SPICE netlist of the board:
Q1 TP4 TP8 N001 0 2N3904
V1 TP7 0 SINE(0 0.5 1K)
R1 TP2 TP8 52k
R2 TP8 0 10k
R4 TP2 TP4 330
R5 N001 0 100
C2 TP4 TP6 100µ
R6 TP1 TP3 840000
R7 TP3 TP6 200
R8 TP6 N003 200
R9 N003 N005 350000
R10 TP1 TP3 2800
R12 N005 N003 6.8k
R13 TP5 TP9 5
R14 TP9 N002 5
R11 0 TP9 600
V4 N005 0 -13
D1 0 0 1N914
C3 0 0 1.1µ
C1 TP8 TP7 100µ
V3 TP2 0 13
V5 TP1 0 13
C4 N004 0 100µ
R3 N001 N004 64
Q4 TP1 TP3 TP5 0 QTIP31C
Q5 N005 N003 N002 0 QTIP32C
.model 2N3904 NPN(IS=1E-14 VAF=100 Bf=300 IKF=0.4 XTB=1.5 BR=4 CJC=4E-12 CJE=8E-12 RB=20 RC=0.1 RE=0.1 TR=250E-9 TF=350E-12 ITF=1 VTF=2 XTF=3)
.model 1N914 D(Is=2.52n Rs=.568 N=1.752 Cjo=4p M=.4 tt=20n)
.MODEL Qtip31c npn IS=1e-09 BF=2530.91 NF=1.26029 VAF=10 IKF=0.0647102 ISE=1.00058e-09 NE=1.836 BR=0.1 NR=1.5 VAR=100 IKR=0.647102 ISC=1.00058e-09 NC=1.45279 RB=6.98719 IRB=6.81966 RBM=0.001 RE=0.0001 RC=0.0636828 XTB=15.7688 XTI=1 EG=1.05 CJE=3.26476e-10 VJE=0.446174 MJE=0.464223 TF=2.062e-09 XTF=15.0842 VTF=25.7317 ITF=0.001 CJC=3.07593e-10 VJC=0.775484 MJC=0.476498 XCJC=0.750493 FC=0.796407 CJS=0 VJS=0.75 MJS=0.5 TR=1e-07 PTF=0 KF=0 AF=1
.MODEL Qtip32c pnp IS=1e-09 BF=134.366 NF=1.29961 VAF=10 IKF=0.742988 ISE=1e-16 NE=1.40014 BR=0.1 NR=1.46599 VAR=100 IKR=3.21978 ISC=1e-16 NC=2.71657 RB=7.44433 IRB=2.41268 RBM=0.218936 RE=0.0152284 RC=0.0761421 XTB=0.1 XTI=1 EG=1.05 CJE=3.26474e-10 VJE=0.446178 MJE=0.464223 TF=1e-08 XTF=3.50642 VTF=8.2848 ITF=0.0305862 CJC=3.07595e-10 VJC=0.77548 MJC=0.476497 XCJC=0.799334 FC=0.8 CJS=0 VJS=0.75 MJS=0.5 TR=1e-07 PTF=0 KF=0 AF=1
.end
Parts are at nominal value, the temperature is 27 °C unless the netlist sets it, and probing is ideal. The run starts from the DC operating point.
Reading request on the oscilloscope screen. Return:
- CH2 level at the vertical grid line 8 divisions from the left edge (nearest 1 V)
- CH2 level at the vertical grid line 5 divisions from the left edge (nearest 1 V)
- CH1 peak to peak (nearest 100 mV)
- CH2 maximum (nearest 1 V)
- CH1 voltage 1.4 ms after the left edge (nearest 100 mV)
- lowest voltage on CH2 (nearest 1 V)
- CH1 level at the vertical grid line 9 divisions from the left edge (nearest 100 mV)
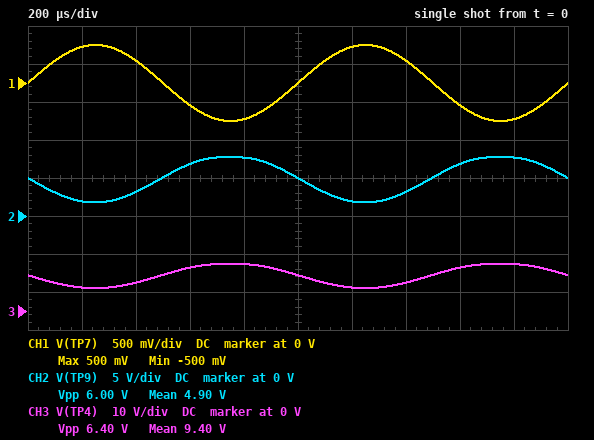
7 V
5 V
1.0 V
8 V
300 mV
2 V
-500 mV
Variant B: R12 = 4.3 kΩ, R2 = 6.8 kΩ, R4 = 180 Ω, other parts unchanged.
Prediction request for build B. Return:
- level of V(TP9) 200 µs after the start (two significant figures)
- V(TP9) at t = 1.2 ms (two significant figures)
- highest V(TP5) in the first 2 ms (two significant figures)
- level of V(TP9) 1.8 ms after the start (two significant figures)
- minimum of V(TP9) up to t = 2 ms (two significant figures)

770 mV
780 mV
3.7 V
3.5 V
690 mV
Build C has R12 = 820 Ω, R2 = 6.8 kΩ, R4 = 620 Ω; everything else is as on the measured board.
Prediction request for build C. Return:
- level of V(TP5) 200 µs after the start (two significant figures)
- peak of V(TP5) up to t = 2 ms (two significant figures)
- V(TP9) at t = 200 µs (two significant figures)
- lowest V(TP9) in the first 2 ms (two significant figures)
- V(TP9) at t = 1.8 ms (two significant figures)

-9.1 V
-3.4 V
-9.4 V
-9.6 V
-4.2 V
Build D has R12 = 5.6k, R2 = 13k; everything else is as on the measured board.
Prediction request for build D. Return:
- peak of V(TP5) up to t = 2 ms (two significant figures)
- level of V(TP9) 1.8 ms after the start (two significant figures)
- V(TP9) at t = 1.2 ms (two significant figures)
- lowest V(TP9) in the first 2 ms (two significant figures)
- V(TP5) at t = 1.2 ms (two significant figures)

7.1 V
6.9 V
910 mV
770 mV
1.0 V
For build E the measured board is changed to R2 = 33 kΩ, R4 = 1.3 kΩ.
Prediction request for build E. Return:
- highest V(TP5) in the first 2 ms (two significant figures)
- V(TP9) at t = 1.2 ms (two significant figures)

12 V
5.2 V
